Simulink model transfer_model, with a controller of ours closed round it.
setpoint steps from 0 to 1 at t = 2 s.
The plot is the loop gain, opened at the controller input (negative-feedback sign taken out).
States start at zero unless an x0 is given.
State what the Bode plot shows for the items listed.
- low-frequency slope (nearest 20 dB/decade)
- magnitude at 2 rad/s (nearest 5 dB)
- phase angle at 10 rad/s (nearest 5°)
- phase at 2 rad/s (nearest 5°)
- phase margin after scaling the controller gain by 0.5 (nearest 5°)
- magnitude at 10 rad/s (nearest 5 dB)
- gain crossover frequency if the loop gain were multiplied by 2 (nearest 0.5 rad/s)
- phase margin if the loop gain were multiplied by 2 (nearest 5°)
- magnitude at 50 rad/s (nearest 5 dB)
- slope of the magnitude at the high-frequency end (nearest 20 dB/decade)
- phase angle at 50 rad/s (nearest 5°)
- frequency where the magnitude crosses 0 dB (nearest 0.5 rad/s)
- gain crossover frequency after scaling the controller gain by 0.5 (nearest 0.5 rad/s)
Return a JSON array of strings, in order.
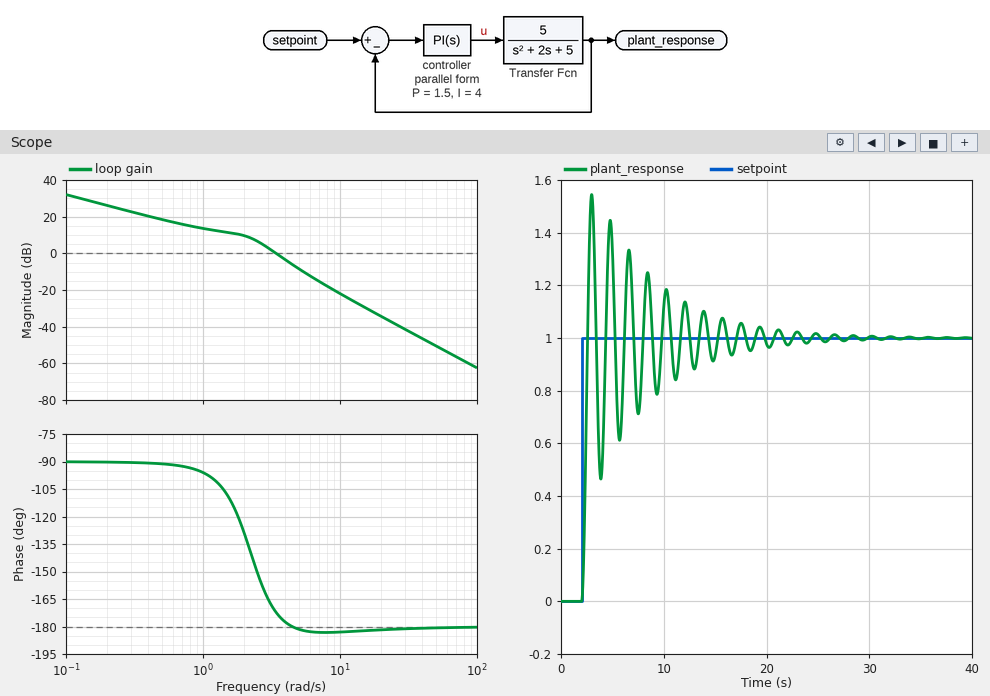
["-20 dB/decade", "10 dB", "-185°", "-130°", "25°", "-20 dB", "4.5 rad/s", "0°", "-50 dB", "-40 dB/decade", "-180°", "3.5 rad/s", "2.5 rad/s"]
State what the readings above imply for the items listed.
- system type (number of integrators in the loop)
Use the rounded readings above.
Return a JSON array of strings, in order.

["1"]
